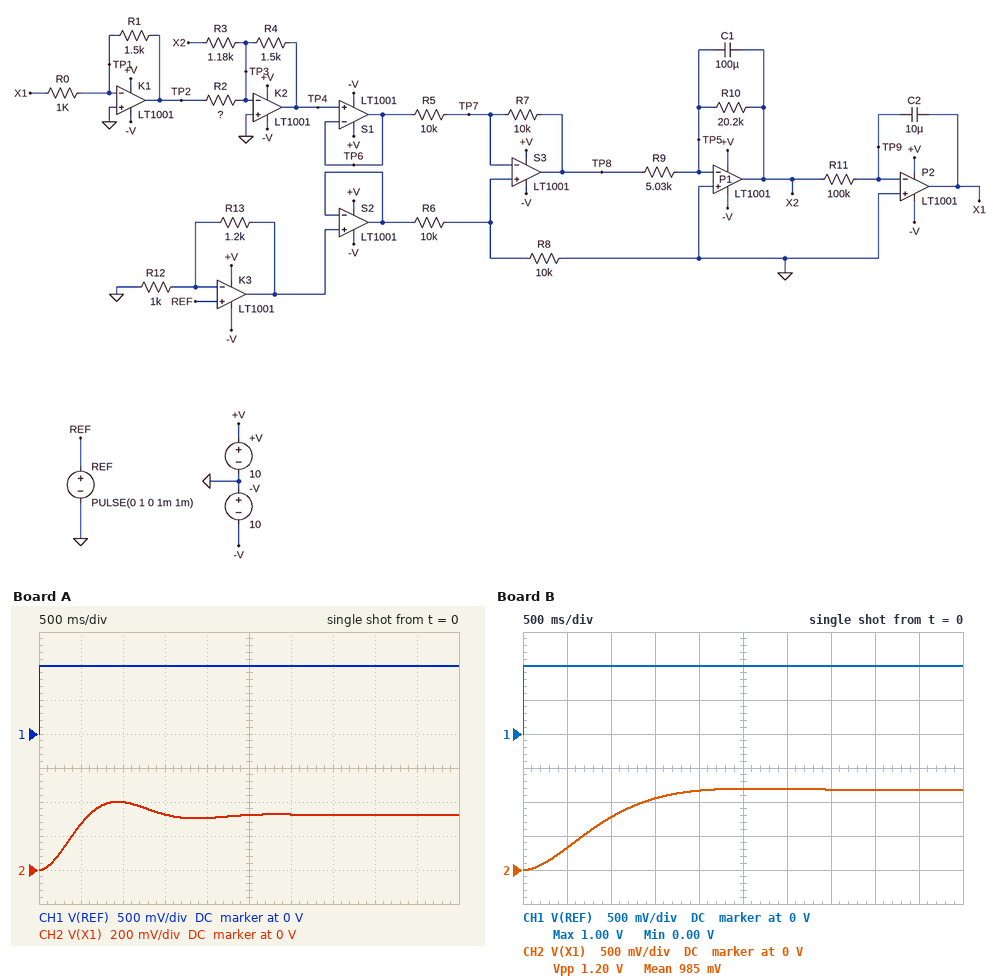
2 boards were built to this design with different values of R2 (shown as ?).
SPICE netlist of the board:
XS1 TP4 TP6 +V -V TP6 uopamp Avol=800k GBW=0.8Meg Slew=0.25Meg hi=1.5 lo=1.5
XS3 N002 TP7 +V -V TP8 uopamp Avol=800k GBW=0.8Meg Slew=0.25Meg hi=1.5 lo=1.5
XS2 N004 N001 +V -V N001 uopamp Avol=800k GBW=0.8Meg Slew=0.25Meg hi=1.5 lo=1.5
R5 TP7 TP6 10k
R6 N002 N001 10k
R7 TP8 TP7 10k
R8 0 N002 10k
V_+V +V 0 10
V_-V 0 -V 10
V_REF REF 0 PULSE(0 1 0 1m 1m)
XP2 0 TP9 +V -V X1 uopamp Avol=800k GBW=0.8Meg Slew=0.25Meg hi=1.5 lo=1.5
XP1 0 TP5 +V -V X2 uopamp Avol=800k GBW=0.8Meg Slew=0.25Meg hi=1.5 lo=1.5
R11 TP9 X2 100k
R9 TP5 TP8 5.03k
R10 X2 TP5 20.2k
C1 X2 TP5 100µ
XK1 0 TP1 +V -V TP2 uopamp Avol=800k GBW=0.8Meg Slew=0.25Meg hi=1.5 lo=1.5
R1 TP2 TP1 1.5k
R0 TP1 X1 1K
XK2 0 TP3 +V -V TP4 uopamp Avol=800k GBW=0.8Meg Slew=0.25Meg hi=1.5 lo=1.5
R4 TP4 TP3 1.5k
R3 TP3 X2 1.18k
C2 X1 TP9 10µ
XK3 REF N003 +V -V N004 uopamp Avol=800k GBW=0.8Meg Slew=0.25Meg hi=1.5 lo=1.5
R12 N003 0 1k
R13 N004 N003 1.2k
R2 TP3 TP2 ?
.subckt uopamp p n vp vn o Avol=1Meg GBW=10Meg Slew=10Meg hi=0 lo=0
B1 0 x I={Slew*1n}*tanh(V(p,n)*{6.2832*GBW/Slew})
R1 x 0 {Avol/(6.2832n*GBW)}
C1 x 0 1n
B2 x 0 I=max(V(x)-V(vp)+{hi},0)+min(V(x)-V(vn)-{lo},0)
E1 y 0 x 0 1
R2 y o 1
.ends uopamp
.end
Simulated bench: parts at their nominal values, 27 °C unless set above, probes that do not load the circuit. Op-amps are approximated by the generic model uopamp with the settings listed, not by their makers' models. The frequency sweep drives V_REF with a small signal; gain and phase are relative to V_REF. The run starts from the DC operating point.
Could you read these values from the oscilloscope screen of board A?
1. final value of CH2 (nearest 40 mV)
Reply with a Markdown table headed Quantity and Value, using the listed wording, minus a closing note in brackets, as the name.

| Quantity | Value |
|---|---|
| final value of CH2 | 320 mV |
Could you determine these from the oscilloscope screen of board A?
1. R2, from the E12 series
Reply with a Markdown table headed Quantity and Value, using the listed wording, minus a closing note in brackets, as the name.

| Quantity | Value |
|---|---|
| R2, from the E12 series | 330 Ω |
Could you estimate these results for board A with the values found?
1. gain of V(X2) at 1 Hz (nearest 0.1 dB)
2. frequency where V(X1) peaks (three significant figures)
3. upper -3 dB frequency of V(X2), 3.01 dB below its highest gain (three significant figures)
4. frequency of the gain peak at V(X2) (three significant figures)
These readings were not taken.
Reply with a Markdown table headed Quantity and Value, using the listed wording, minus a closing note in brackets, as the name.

| Quantity | Value |
|---|---|
| gain of V(X2) at 1 Hz | -1.4 dB |
| frequency where V(X1) peaks | 477 mHz |
| upper -3 dB frequency of V(X2), 3.01 dB below its highest gain | 874 mHz |
| frequency of the gain peak at V(X2) | 586 mHz |
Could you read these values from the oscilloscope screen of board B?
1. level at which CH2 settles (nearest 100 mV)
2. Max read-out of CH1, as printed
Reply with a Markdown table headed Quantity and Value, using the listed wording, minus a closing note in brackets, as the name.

| Quantity | Value |
|---|---|
| level at which CH2 settles | 1.2 V |
| Max read-out of CH1, as printed | 1.00 V |
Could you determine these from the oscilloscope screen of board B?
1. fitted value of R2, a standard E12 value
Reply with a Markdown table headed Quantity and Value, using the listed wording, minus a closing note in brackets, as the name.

| Quantity | Value |
|---|---|
| fitted value of R2, a standard E12 value | 1.2 kΩ |
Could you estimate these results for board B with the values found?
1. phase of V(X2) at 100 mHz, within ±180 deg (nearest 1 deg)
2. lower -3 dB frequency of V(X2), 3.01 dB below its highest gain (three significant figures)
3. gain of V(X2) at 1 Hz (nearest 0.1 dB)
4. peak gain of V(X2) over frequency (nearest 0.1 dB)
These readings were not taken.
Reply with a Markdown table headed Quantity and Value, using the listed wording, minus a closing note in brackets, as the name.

| Quantity | Value |
|---|---|
| phase of V(X2) at 100 mHz, within ±180 deg | -120 deg |
| lower -3 dB frequency of V(X2), 3.01 dB below its highest gain | 150 mHz |
| gain of V(X2) at 1 Hz | -3.4 dB |
| peak gain of V(X2) over frequency | 3.2 dB |
